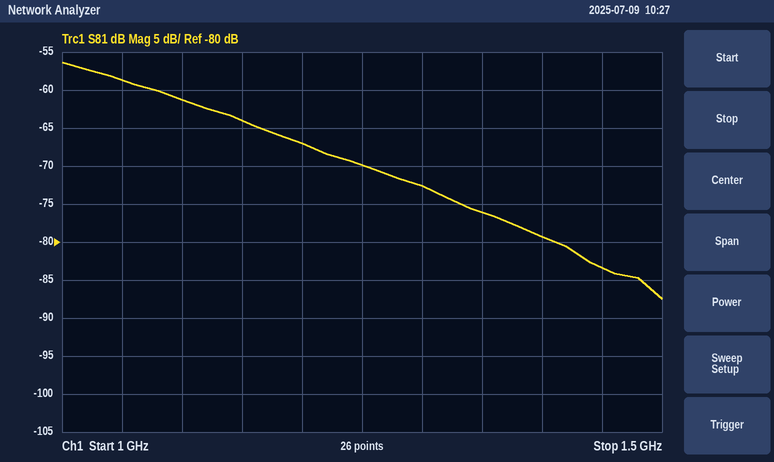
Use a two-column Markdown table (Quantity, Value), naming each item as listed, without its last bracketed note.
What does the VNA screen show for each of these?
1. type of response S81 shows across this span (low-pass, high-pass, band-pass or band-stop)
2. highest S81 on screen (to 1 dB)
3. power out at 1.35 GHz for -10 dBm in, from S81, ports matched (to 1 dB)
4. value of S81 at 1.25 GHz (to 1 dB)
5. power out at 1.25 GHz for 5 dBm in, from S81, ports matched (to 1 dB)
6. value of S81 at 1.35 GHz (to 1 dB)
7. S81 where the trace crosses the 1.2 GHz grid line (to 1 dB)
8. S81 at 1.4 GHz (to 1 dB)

| Quantity | Value |
|---|---|
| type of response S81 shows across this span | low-pass |
| highest S81 on screen | -56 dB |
| power out at 1.35 GHz for -10 dBm in, from S81, ports matched | -86 dBm |
| value of S81 at 1.25 GHz | -70 dB |
| power out at 1.25 GHz for 5 dBm in, from S81, ports matched | -65 dBm |
| value of S81 at 1.35 GHz | -76 dB |
| S81 where the trace crosses the 1.2 GHz grid line | -67 dB |
| S81 at 1.4 GHz | -79 dB |
